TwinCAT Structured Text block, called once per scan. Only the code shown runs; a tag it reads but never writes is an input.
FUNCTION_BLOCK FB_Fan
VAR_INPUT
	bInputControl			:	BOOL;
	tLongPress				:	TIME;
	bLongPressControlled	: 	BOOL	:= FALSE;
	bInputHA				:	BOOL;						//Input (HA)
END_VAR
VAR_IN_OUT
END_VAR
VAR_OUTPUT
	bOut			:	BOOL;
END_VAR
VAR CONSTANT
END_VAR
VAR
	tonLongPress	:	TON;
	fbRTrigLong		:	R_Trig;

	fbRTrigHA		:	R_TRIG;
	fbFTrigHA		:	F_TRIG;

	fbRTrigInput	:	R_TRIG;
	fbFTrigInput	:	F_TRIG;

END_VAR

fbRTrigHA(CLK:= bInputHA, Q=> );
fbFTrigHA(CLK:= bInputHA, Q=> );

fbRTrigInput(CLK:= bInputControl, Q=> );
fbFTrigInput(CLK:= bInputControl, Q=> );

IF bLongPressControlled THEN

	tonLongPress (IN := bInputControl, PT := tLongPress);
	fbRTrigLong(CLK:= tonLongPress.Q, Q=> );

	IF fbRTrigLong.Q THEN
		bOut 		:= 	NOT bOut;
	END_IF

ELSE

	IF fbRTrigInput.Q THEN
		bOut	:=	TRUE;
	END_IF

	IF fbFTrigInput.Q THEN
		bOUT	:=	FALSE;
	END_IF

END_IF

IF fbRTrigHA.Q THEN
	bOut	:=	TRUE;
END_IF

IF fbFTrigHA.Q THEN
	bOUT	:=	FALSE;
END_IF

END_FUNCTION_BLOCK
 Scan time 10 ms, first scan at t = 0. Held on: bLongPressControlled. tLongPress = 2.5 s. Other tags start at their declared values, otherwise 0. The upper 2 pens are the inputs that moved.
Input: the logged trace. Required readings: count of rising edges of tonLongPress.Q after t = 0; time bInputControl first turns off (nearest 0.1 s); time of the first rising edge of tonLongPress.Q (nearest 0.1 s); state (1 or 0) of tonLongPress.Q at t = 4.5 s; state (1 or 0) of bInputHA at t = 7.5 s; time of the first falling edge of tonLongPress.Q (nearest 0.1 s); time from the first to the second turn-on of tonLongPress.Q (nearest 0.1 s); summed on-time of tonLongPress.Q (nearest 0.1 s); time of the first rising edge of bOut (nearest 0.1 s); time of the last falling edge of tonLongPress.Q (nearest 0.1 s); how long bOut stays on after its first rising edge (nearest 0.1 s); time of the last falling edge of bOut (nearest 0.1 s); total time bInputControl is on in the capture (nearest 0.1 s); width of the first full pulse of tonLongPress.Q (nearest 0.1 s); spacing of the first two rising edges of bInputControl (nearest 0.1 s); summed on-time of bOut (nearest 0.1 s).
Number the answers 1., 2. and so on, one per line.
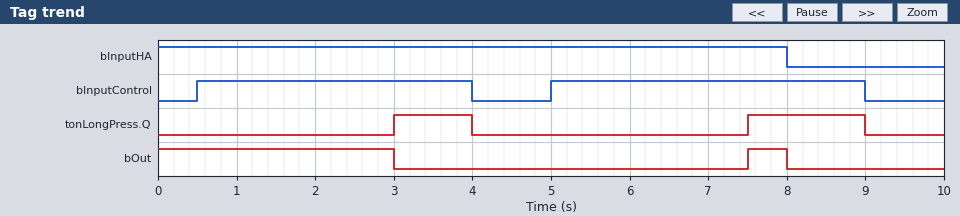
1. 2
2. 4.0 s
3. 3.0 s
4. 0
5. 1
6. 4.0 s
7. 4.5 s
8. 2.5 s
9. 7.5 s
10. 9.0 s
11. 0.5 s
12. 8.0 s
13. 7.5 s
14. 1.0 s
15. 4.5 s
16. 3.5 s
